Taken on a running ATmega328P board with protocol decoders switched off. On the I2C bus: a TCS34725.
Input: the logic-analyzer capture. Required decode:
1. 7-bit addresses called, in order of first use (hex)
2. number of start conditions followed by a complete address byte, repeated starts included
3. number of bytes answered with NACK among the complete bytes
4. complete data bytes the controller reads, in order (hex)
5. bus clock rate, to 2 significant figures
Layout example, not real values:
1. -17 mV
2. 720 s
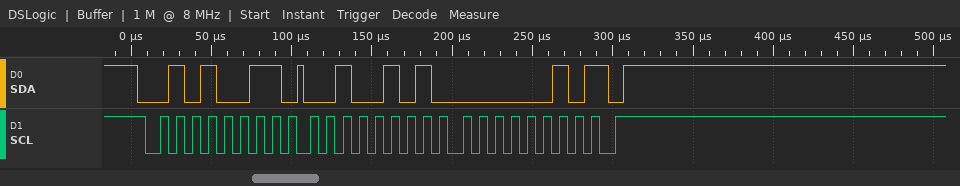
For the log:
1. 0x29
2. 1
3. 1
4. 25 02
5. 100 kHz
